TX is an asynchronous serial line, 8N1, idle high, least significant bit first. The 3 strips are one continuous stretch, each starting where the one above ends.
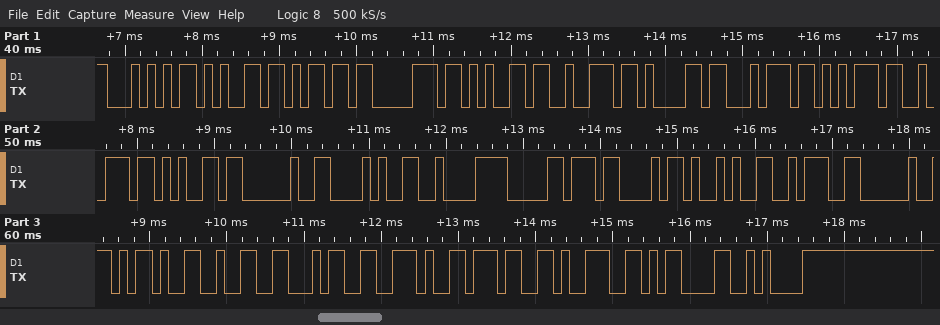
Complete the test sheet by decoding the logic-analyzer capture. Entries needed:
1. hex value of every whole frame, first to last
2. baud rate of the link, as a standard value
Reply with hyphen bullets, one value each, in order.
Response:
- 54 65 6D 70 65 72 61 74 75 72 65 20 28 C2 B0 43 29 3A 20 2D 32 34 2E 37 39 0D 0A
- 9600 baud
